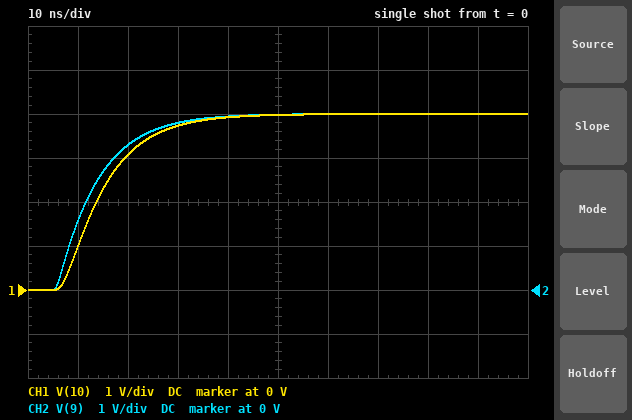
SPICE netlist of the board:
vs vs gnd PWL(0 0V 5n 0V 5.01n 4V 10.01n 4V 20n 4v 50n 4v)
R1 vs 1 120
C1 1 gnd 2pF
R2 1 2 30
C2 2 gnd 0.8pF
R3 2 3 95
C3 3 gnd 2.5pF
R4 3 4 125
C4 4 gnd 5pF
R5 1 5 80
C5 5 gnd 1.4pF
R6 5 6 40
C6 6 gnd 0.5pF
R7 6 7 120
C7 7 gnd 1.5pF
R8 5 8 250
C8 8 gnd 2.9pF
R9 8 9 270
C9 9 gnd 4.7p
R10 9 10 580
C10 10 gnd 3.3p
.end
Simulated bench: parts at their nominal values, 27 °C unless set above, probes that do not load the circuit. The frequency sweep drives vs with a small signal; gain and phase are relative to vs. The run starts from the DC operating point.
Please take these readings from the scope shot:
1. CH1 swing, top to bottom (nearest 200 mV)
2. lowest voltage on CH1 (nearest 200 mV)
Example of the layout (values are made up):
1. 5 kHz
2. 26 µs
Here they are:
1. 4.0 V
2. 0 V
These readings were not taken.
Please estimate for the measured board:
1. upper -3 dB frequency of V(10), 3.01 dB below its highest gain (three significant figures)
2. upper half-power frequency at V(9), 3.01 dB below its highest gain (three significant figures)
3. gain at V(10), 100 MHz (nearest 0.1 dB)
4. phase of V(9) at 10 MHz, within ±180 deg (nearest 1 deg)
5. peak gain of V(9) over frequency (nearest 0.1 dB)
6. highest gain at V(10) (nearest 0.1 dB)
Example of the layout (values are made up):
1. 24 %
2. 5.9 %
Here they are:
1. 18.6 MHz
2. 19.5 MHz
3. -19.1 dB
4. -30 deg
5. 0 dB
6. 0 dB
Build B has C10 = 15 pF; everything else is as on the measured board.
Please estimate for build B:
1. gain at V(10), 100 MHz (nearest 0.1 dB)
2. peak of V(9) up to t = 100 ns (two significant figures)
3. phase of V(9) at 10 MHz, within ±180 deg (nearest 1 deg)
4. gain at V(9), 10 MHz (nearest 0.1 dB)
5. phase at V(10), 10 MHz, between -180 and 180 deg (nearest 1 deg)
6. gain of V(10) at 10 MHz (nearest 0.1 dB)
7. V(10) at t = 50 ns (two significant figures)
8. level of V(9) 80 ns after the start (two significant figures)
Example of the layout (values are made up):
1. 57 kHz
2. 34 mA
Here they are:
1. -30.1 dB
2. 4.0 V
3. -39 deg
4. -3.7 dB
5. -68 deg
6. -4.9 dB
7. 3.4 V
8. 3.9 V
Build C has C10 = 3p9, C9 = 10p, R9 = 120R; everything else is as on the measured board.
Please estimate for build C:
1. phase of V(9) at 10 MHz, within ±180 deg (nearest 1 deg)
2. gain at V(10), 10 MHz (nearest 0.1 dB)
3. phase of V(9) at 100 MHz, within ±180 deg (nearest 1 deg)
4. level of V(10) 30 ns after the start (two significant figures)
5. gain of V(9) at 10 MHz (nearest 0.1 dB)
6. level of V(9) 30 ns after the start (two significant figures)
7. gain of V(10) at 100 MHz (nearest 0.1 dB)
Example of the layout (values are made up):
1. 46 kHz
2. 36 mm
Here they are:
1. -36 deg
2. -1.6 dB
3. -109 deg
4. 3.5 V
5. -1.5 dB
6. 3.6 V
7. -22.1 dB
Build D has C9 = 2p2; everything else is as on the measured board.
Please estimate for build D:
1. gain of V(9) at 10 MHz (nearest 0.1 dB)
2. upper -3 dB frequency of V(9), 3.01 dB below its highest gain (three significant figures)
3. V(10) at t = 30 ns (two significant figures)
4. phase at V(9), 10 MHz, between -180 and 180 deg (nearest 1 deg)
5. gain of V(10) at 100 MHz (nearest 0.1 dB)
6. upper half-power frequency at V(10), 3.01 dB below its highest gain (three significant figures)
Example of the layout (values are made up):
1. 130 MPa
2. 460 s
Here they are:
1. -0.7 dB
2. 23.9 MHz
3. 3.9 V
4. -25 deg
5. -16.8 dB
6. 22.3 MHz
